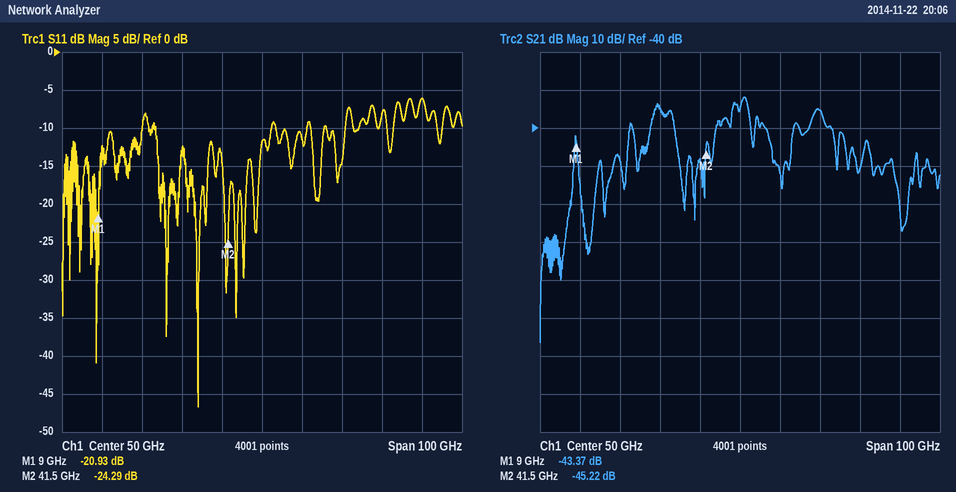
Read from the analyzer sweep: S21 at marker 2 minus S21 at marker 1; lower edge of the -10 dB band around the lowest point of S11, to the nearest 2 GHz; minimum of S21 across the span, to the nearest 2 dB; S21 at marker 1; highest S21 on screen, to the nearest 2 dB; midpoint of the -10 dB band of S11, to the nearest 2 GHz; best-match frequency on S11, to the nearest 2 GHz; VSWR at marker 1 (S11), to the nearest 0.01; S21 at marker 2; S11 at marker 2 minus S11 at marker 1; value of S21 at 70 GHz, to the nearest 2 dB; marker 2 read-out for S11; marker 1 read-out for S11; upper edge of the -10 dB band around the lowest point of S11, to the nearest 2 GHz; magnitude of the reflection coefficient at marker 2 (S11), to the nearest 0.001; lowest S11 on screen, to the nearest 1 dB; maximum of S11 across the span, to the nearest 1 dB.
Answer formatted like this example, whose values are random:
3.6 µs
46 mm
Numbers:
-1.85 dB
24 GHz
-96 dB
-43.37 dB
-32 dB
38 GHz
34 GHz
1.20
-45.22 dB
-3.36 dB
-36 dB
-24.29 dB
-20.93 dB
52 GHz
0.061
-47 dB
-6 dB
